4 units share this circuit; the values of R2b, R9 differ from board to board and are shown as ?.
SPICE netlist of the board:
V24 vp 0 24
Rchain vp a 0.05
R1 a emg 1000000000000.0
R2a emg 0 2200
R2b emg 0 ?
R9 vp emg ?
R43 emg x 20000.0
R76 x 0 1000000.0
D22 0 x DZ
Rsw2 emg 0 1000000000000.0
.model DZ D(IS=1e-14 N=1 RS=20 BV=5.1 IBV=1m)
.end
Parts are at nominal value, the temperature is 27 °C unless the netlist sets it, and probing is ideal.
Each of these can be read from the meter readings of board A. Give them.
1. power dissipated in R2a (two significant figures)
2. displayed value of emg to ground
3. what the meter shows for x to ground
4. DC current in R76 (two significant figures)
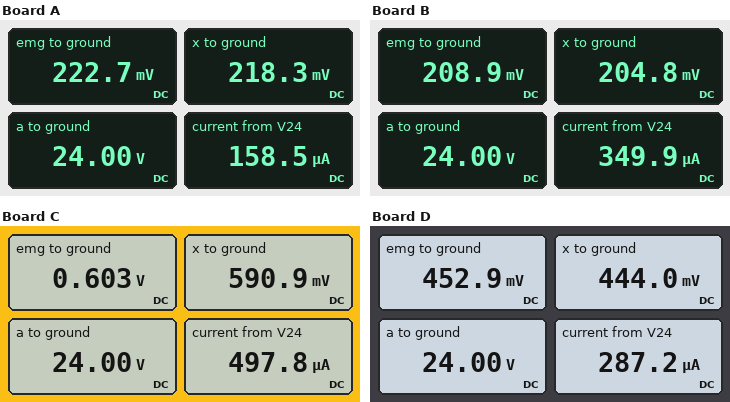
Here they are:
23 µW
222.7 mV
218.3 mV
220 nA
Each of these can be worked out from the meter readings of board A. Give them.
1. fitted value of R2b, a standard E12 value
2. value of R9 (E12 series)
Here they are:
3.9 kΩ
150 kΩ
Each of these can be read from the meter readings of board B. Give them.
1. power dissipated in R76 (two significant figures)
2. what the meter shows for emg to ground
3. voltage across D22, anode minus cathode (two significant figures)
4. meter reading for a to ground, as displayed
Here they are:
42 nW
208.9 mV
-200 mV
24.00 V
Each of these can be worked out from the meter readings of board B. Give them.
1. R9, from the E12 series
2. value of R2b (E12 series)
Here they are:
68 kΩ
820 Ω
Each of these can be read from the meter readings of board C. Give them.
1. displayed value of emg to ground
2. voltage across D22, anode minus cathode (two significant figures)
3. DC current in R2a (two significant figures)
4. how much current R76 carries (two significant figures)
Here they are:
0.603 V
-590 mV
270 µA
590 nA
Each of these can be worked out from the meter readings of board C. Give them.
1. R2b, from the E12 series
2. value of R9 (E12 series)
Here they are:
2.7 kΩ
47 kΩ
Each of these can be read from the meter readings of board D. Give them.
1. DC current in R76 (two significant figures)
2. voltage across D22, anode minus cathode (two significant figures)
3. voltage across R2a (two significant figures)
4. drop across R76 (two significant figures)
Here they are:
440 nA
-440 mV
450 mV
440 mV
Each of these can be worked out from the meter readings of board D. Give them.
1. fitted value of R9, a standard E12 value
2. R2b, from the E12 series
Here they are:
82 kΩ
5.6 kΩ
